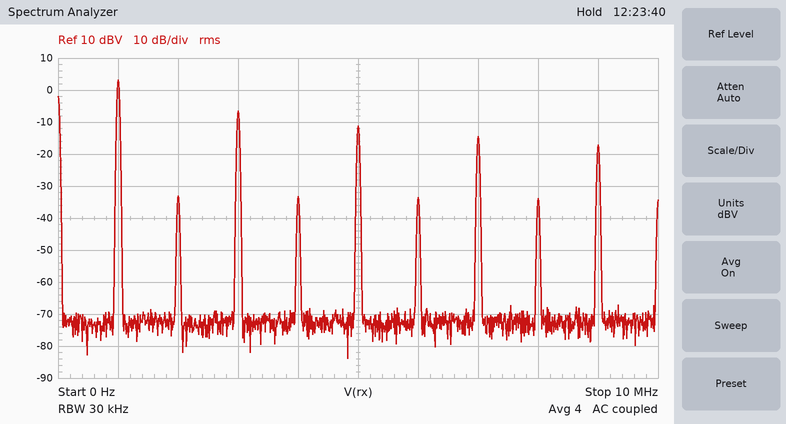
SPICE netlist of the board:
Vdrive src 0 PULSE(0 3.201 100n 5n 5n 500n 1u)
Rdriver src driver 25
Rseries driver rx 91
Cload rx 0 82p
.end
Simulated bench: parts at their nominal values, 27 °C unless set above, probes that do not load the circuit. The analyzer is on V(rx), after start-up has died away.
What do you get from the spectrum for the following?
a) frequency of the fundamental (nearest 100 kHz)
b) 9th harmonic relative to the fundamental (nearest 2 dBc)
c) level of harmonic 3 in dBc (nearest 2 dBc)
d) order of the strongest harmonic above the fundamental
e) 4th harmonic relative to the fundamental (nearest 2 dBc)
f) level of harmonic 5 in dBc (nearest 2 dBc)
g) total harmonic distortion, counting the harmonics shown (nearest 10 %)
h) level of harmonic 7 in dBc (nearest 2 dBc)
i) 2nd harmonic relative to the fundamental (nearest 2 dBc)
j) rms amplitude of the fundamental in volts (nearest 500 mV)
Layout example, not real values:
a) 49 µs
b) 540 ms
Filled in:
a) 1.0 MHz
b) -20 dBc
c) -10 dBc
d) 3
e) -36 dBc
f) -14 dBc
g) 40 %
h) -18 dBc
i) -36 dBc
j) 1.5 V
